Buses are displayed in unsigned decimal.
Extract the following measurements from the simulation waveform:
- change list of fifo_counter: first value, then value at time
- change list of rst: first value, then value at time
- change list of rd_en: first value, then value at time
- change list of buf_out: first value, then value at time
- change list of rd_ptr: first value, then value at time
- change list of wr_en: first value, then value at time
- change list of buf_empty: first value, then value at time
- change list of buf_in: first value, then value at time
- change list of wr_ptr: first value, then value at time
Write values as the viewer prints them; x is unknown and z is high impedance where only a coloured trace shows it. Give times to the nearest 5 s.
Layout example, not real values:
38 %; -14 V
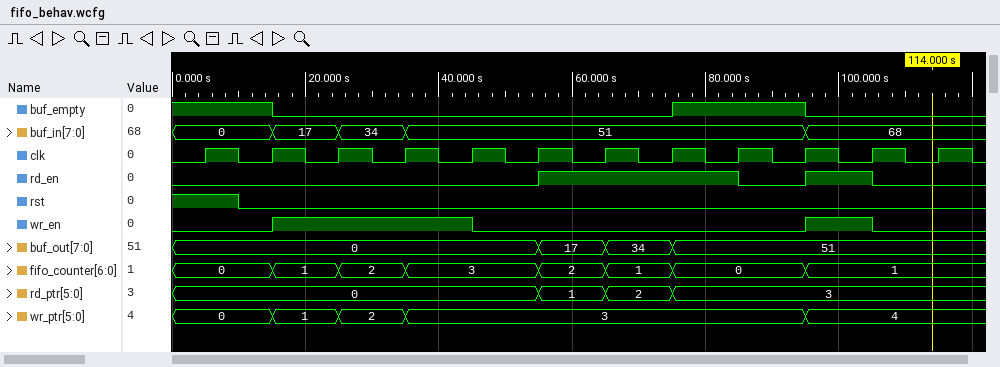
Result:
0, 1 at 15 s, 2 at 25 s, 3 at 35 s, 2 at 55 s, 1 at 65 s, 0 at 75 s, 1 at 95 s; 1, 0 at 10 s; 0, 1 at 55 s, 0 at 85 s, 1 at 95 s, 0 at 105 s; 0, 17 at 55 s, 34 at 65 s, 51 at 75 s; 0, 1 at 55 s, 2 at 65 s, 3 at 75 s; 0, 1 at 15 s, 0 at 45 s, 1 at 95 s, 0 at 105 s; 1, 0 at 15 s, 1 at 75 s, 0 at 95 s; 0, 17 at 15 s, 34 at 25 s, 51 at 35 s, 68 at 95 s; 0, 1 at 15 s, 2 at 25 s, 3 at 35 s, 4 at 95 s
